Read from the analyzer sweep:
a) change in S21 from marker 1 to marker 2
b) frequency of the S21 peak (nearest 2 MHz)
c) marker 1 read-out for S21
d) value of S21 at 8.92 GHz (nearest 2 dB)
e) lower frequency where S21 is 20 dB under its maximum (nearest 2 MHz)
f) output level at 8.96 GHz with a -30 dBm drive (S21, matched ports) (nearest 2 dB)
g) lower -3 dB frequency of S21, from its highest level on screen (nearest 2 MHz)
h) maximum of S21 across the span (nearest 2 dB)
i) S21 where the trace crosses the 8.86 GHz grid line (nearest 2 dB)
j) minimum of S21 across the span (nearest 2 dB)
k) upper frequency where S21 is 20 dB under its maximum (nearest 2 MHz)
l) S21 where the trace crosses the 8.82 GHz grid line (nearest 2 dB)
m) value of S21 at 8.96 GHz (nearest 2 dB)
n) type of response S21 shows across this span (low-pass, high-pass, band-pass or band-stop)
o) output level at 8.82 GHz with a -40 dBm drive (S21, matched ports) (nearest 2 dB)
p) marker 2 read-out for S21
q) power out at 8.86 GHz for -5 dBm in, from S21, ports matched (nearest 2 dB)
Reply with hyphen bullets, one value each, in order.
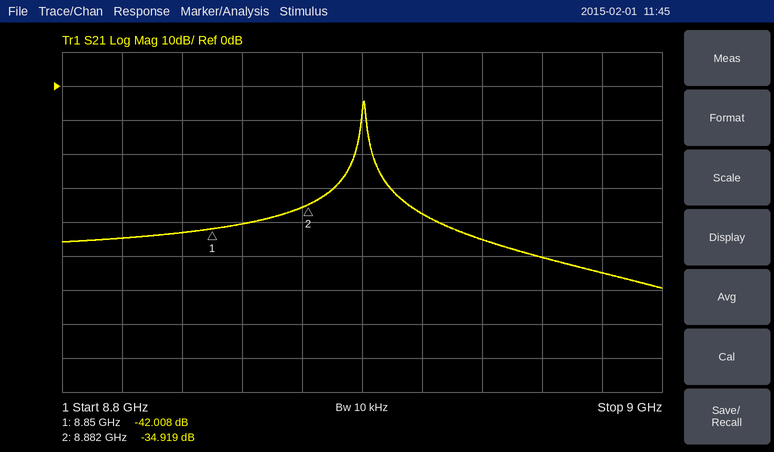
- 7.089 dB
- 8.900 GHz
- -42.008 dB
- -38 dB
- 8.896 GHz
- -80 dBm
- 8.900 GHz
- -4 dB
- -40 dB
- -60 dB
- 8.906 GHz
- -44 dB
- -50 dB
- band-pass
- -84 dBm
- -34.919 dB
- -46 dBm
